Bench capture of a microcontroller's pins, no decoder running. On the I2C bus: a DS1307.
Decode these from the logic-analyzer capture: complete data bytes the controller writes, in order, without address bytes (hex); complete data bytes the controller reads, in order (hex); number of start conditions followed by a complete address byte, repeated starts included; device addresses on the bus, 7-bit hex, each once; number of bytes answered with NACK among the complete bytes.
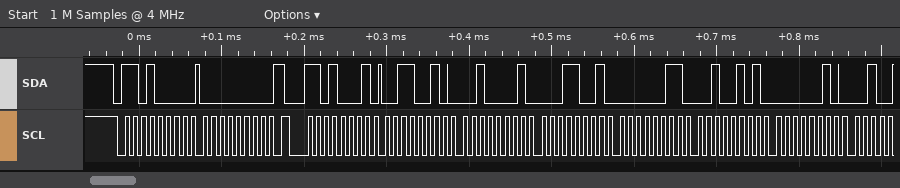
00
32 21 19 03 25 02
2
0x68
0
